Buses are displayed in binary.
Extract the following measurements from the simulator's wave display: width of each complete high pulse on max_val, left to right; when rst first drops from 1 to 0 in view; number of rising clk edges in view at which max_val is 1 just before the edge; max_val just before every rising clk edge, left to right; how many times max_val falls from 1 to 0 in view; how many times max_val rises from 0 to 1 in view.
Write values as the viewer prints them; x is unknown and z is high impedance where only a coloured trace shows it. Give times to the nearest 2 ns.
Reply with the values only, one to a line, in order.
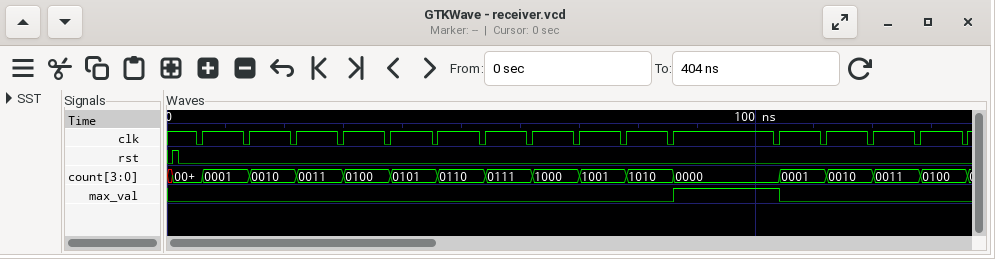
18 ns
2 ns
1
0 0 0 0 0 0 0 0 0 0 0 1 0 0 0 0
1
1
